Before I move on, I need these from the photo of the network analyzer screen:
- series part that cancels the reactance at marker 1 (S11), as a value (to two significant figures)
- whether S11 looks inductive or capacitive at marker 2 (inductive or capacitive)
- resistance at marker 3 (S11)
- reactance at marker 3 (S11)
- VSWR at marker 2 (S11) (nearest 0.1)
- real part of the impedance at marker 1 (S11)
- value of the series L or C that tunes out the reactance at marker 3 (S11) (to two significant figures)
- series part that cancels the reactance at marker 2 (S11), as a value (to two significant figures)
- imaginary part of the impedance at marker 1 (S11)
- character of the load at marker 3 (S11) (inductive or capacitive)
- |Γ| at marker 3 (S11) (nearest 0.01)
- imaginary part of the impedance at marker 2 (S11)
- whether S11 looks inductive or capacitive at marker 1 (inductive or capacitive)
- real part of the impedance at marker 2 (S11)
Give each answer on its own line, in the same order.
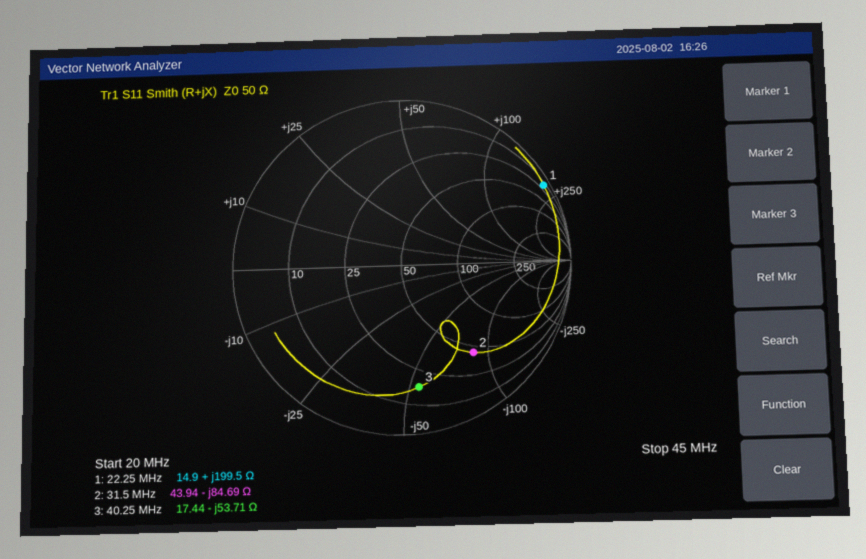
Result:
36 pF
capacitive
17.44 Ω
-53.71 Ω
5.1
14.9 Ω
210 nH
430 nH
+199.5 Ω
capacitive
0.73
-84.69 Ω
inductive
43.94 Ω
